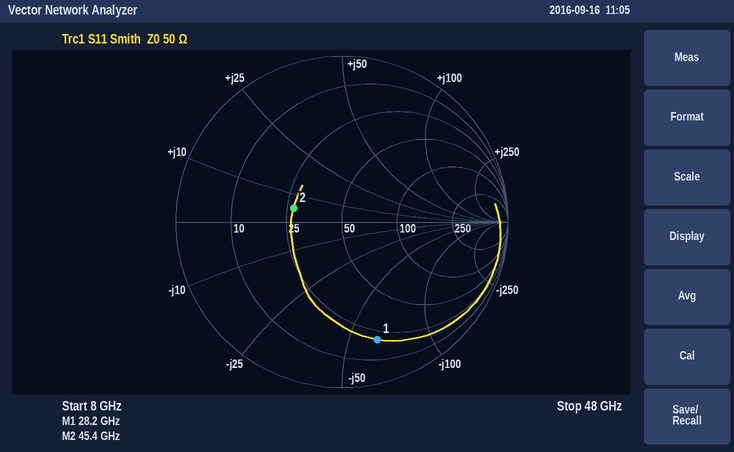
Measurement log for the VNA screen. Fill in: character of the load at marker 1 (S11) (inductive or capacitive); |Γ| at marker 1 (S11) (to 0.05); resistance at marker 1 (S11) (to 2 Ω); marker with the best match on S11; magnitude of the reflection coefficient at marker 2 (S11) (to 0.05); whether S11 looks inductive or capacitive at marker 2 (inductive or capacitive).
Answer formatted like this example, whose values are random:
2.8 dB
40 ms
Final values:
capacitive
0.75
20 Ω
marker 2
0.30
inductive
